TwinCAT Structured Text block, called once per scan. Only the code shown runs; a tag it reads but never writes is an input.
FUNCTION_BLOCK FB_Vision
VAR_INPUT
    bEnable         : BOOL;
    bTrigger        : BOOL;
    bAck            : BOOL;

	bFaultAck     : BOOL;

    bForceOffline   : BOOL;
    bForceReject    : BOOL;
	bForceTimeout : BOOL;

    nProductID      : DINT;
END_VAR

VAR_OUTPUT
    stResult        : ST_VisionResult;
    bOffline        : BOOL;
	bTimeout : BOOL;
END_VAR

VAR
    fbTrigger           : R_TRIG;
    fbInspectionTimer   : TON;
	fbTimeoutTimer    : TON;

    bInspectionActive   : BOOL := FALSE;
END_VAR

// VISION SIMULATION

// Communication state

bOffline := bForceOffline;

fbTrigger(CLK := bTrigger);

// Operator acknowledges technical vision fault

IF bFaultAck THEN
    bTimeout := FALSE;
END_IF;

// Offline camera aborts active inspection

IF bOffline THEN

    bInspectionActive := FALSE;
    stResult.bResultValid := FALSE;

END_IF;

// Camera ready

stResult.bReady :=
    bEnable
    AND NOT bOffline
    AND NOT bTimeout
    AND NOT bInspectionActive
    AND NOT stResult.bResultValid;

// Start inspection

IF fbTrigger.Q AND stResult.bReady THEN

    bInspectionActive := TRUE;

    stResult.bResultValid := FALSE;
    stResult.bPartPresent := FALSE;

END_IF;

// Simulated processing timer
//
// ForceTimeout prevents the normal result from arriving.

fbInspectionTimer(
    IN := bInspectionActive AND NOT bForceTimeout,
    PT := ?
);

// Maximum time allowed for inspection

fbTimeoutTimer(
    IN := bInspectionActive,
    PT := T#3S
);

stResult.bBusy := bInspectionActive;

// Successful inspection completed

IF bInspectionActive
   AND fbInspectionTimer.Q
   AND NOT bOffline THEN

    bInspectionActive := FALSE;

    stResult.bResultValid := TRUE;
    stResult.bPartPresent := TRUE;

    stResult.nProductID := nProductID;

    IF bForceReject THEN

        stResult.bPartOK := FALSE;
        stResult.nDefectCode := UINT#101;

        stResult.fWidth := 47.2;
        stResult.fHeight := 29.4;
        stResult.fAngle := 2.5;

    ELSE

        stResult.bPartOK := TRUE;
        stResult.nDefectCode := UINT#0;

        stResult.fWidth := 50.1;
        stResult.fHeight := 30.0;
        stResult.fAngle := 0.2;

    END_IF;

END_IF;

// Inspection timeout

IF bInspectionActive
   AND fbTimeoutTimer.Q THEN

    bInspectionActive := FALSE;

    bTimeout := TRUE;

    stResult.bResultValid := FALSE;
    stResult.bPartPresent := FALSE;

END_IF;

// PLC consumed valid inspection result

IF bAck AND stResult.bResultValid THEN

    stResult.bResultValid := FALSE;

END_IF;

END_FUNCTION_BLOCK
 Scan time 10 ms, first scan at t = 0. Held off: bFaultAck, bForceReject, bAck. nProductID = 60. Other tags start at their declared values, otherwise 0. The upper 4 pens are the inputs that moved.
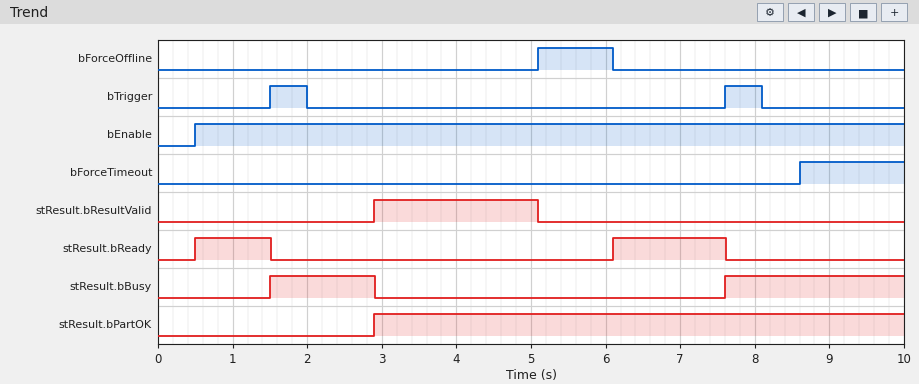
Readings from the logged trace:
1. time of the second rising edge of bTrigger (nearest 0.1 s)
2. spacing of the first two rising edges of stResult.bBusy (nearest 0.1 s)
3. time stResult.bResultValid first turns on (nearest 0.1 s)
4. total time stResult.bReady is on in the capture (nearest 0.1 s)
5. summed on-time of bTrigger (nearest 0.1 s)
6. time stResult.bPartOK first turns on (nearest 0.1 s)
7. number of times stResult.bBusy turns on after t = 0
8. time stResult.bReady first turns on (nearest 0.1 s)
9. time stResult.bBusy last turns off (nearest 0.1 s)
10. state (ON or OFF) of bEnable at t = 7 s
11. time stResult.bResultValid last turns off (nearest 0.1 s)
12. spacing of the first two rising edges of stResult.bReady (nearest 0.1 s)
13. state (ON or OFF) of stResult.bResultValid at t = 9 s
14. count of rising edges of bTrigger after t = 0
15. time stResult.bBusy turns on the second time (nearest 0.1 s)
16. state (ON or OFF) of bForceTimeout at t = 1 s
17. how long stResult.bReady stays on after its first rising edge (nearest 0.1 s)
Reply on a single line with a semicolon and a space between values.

7.6 s; 6.1 s; 2.9 s; 2.5 s; 1.0 s; 2.9 s; 2; 0.5 s; 2.9 s; ON; 5.1 s; 5.6 s; OFF; 2; 7.6 s; OFF; 1.0 s
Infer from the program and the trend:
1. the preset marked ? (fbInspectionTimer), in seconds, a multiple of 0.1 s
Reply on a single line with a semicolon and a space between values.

1.4 s
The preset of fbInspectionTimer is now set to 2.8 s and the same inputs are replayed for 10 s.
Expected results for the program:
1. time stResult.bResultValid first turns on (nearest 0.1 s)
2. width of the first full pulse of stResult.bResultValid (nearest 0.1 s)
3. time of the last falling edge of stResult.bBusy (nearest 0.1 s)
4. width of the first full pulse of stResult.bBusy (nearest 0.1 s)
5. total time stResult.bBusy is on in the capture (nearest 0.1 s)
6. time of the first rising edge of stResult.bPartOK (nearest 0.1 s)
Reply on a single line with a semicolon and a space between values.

4.3 s; 0.8 s; 4.3 s; 2.8 s; 5.2 s; 4.3 s
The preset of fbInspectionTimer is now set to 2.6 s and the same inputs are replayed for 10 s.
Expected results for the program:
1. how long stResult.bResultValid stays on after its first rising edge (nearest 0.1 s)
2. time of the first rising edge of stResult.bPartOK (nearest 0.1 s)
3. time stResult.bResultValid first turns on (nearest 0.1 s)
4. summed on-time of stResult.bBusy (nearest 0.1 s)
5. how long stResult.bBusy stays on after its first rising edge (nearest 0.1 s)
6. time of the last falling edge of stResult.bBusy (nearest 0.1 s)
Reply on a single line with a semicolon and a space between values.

1.0 s; 4.1 s; 4.1 s; 5.0 s; 2.6 s; 4.1 s
